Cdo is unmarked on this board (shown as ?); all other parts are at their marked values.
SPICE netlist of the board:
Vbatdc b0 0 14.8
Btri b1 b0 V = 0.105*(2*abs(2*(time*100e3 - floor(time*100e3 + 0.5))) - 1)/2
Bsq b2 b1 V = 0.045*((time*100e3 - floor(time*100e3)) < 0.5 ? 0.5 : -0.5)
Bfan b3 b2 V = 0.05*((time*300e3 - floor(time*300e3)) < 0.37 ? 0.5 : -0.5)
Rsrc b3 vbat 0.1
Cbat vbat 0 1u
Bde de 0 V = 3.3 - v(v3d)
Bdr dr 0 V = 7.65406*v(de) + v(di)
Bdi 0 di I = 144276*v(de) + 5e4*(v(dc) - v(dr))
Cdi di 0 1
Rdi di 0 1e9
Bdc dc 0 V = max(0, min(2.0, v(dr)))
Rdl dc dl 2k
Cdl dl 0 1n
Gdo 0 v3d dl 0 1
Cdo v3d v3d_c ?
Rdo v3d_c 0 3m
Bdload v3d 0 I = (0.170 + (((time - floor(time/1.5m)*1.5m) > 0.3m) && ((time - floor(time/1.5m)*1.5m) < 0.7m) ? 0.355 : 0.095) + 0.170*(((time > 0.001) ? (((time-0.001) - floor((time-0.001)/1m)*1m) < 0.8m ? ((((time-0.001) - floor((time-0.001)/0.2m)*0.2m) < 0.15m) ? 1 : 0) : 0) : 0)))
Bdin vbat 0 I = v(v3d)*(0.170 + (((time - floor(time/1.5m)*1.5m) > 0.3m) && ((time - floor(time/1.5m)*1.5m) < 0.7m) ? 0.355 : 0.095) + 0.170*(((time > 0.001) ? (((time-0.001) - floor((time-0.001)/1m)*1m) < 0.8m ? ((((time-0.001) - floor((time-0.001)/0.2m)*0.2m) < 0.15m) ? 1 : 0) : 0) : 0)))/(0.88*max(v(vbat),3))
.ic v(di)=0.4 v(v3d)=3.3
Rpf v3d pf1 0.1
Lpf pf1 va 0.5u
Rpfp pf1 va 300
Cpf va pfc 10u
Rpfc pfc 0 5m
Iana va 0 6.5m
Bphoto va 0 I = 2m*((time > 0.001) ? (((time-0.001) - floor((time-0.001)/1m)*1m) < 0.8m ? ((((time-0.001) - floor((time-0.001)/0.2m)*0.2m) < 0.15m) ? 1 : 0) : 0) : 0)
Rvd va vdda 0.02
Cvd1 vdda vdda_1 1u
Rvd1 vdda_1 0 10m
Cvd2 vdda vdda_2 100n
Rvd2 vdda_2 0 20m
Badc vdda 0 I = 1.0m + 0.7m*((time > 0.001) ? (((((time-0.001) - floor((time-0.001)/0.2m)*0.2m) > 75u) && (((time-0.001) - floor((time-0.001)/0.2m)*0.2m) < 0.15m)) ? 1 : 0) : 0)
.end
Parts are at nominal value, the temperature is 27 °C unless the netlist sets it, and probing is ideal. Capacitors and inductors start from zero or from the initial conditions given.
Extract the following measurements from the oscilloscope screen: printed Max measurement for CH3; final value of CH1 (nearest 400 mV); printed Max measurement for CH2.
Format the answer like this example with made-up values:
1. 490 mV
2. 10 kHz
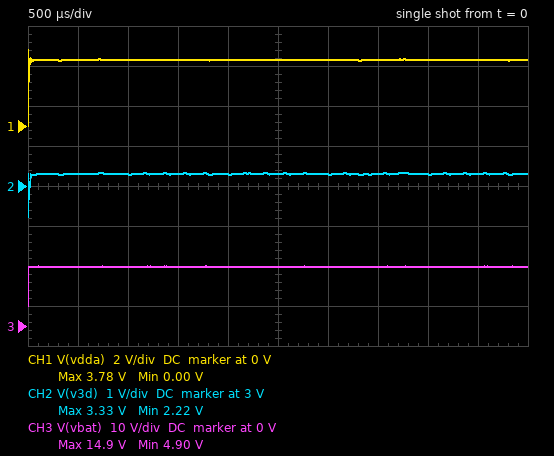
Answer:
1. 14.9 V
2. 3.2 V
3. 3.33 V
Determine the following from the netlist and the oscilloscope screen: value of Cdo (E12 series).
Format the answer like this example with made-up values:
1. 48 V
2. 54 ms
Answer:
1. 33 µF
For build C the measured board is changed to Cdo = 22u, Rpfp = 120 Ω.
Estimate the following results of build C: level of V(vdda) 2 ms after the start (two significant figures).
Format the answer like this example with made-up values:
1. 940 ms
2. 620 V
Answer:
1. 3.3 V
